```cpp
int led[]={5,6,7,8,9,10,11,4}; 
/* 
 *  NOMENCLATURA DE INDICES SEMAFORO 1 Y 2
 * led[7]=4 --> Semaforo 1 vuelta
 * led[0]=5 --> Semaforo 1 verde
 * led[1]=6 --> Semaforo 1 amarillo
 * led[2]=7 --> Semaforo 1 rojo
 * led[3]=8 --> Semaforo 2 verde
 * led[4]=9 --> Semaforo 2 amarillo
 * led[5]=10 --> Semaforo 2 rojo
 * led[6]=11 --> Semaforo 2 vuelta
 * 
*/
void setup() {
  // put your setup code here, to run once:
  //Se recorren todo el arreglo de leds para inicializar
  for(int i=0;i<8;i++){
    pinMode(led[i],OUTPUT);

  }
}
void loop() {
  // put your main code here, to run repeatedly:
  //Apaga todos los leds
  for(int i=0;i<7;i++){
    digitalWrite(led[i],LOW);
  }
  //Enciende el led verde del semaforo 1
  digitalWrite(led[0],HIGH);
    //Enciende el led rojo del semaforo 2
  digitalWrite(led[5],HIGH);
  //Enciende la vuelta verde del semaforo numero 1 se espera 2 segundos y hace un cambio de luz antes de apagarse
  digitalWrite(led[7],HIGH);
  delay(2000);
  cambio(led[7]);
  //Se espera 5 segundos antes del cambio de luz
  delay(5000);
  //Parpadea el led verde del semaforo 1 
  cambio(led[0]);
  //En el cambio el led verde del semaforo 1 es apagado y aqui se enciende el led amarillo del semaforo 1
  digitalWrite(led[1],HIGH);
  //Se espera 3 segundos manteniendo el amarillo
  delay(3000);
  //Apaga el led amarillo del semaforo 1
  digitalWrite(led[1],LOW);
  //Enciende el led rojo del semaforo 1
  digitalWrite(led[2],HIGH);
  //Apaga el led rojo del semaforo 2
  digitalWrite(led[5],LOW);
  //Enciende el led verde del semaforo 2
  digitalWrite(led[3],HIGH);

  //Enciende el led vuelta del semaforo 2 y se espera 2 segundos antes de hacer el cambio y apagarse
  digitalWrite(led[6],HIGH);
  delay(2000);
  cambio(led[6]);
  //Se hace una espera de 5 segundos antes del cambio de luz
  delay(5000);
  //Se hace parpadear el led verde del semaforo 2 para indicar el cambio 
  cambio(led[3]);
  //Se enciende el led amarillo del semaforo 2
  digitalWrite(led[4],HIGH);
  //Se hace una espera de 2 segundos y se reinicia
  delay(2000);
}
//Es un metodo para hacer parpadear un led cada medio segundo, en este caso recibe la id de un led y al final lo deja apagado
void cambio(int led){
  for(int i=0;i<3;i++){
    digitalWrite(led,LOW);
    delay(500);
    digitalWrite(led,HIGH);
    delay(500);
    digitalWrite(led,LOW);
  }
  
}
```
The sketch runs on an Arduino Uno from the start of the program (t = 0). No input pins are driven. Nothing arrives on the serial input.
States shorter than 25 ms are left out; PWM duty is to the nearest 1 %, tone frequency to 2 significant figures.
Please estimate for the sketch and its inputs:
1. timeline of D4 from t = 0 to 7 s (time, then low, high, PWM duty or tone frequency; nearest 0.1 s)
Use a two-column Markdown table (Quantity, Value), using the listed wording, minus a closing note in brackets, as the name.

| Quantity | Value |
|---|---|
| timeline of D4 from t = 0 to 7 s | 0 s high; 2 s low; 2.5 s high; 3 s low; 3.5 s high; 4 s low; 4.5 s high; 5 s low |
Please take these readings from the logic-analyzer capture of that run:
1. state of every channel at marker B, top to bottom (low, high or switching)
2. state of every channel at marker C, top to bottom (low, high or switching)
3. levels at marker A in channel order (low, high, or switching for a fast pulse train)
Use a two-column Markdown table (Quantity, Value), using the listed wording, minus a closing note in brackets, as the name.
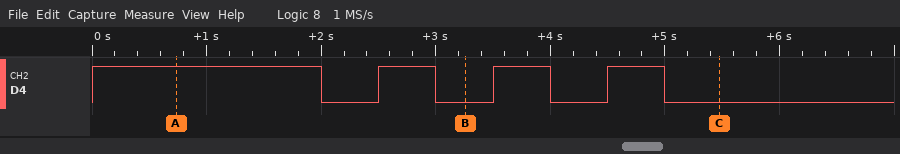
| Quantity | Value |
|---|---|
| state of every channel at marker B, top to bottom | D4 low |
| state of every channel at marker C, top to bottom | D4 low |
| levels at marker A in channel order | D4 high |
